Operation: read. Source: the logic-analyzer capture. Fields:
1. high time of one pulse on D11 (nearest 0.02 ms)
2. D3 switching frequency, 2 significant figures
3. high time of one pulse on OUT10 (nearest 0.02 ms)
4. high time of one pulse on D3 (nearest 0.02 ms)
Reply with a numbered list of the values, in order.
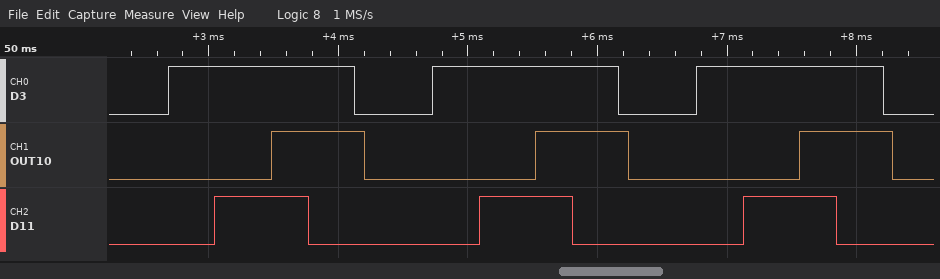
1. 0.72 ms
2. 490 Hz
3. 0.72 ms
4. 1.44 ms
